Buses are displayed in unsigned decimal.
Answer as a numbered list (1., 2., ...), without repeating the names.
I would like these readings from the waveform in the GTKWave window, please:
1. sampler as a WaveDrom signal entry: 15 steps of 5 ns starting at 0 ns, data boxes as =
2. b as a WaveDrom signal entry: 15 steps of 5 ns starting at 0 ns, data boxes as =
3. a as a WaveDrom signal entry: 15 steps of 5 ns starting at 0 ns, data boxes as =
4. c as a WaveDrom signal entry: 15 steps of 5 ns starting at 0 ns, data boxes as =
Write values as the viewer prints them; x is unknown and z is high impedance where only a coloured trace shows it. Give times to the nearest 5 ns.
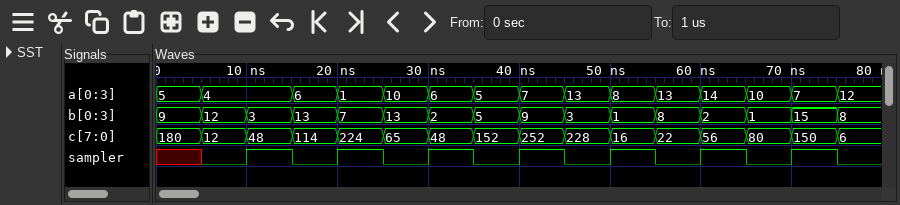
1. {name: 'sampler', wave: 'x01010101010101'}
2. {name: 'b', wave: '===============', data: '9 12 3 13 7 13 2 5 9 3 1 8 2 1 15'}
3. {name: 'a', wave: '==.============', data: '5 4 6 1 10 6 5 7 13 8 13 14 10 7'}
4. {name: 'c', wave: '===============', data: '180 12 48 114 224 65 48 152 252 228 16 22 56 80 150'}
